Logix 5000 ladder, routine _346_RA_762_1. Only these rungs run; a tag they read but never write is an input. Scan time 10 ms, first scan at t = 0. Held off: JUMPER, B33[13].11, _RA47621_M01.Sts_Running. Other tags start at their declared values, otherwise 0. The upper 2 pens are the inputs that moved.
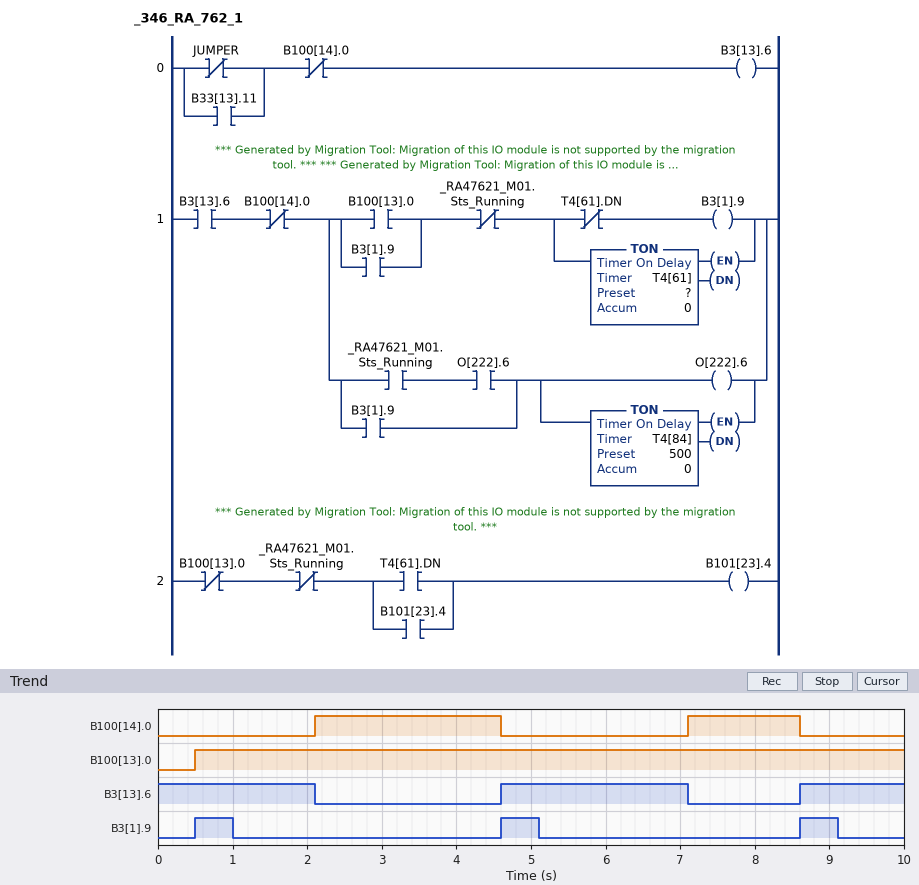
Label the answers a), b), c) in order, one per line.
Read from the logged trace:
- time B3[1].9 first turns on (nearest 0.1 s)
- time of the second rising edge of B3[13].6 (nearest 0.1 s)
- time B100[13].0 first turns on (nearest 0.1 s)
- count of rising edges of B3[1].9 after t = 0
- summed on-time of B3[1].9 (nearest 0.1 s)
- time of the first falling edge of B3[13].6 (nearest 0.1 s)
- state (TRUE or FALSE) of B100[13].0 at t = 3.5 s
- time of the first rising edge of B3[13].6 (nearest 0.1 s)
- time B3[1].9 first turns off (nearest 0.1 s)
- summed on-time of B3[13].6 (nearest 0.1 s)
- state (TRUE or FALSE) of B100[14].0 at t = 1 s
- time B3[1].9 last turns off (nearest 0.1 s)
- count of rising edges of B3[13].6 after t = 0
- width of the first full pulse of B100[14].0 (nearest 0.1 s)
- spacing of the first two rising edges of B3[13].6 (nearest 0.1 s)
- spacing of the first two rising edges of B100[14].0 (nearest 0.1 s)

a) 0.5 s
b) 8.6 s
c) 0.5 s
d) 3
e) 1.5 s
f) 2.1 s
g) TRUE
h) 4.6 s
i) 1.0 s
j) 6.0 s
k) FALSE
l) 9.1 s
m) 2
n) 2.5 s
o) 4.0 s
p) 5.0 s
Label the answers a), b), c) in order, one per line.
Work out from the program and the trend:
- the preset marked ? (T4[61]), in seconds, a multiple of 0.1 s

a) 0.5 s
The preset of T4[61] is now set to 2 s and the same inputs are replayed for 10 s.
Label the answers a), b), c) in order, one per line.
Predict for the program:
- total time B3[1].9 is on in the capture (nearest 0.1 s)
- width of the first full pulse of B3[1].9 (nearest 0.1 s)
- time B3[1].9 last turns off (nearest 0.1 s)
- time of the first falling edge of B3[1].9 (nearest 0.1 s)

a) 5.0 s
b) 1.6 s
c) 6.6 s
d) 2.1 s
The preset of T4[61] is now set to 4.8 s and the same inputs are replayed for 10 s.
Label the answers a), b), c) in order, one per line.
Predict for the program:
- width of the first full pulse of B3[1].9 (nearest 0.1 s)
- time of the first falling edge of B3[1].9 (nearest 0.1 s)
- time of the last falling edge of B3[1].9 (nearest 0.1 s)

a) 1.6 s
b) 2.1 s
c) 7.1 s
